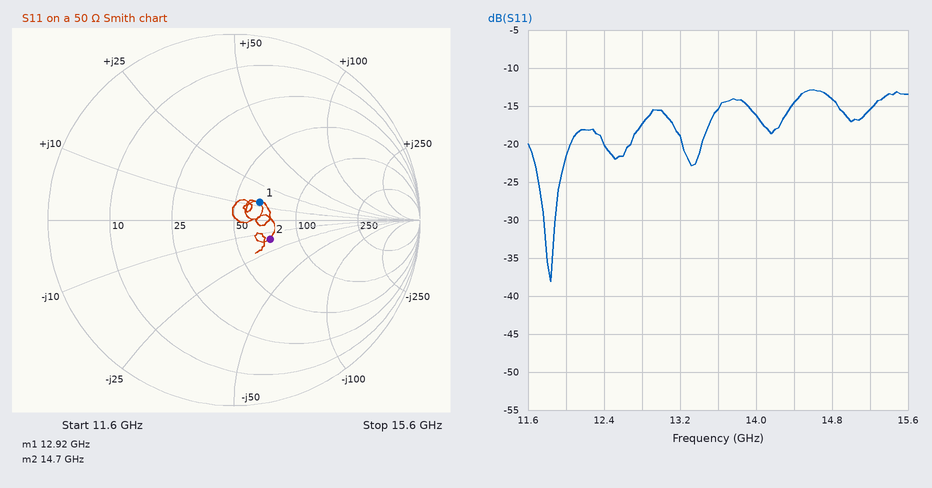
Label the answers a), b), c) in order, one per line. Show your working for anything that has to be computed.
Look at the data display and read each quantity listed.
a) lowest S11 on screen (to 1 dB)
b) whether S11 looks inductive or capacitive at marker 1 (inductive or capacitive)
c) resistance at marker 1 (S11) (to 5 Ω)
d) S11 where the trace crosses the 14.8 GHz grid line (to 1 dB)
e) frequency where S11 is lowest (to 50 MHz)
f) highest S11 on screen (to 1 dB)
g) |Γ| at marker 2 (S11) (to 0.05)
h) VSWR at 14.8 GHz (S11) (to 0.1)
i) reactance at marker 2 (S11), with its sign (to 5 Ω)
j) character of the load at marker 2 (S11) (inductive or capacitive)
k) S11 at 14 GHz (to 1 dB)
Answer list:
a) -38 dB
b) inductive
c) 65 Ω
d) -14 dB
e) 11.85 GHz
f) -13 dB
g) 0.20
h) |Γ| = 10^(-14/20) = 0.1995; VSWR = (1 + 0.1995)/(1 − 0.1995) ≈ 1.5
i) -15 Ω
j) capacitive
k) -16 dB
